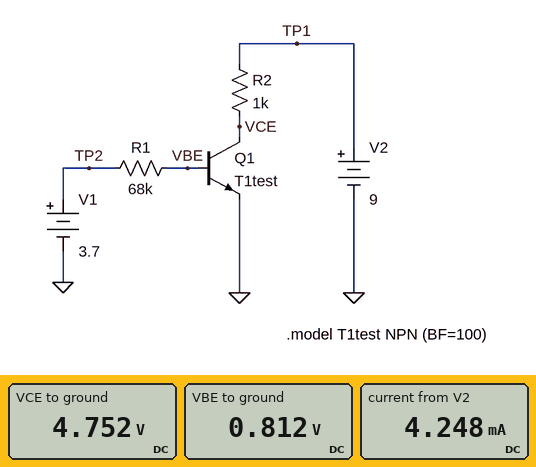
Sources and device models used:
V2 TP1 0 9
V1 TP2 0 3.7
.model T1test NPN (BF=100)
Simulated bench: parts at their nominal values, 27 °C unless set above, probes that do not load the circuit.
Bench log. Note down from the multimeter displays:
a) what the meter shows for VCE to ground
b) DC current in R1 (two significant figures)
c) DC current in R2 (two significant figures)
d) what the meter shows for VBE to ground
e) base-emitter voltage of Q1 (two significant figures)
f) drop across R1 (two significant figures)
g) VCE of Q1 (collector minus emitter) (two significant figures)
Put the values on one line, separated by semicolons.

4.752 V; 42 µA; 4.2 mA; 0.812 V; 810 mV; 2.9 V; 4.8 V
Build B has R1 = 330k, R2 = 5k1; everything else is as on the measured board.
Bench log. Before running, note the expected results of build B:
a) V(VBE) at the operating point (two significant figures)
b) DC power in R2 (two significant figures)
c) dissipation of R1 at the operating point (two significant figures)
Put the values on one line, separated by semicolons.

770 mV; 4.0 mW; 26 µW
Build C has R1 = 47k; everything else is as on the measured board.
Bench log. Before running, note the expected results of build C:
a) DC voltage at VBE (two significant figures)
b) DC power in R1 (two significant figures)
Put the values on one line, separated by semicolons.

820 mV; 180 µW
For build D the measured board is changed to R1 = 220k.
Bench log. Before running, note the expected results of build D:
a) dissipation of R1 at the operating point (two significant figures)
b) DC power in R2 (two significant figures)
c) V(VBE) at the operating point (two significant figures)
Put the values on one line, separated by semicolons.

39 µW; 1.8 mW; 780 mV
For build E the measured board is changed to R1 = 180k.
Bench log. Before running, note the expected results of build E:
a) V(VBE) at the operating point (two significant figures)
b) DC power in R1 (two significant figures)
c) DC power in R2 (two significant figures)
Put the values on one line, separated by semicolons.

790 mV; 47 µW; 2.6 mW
